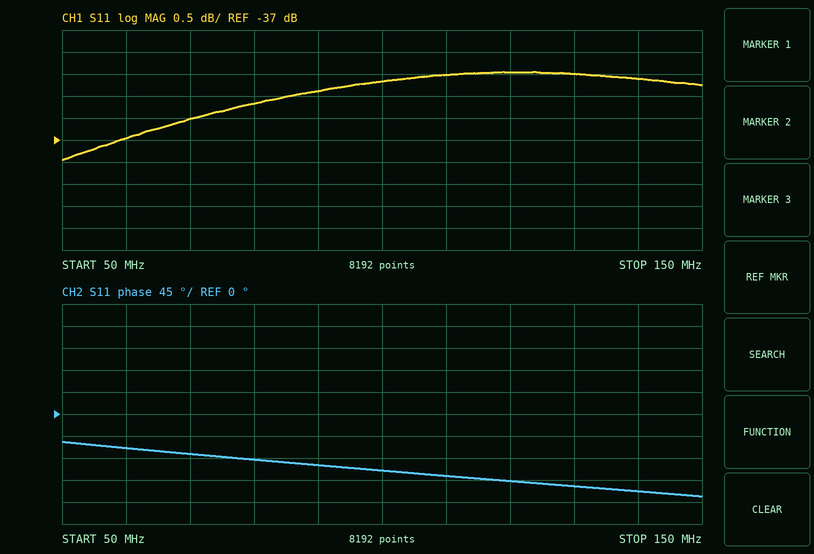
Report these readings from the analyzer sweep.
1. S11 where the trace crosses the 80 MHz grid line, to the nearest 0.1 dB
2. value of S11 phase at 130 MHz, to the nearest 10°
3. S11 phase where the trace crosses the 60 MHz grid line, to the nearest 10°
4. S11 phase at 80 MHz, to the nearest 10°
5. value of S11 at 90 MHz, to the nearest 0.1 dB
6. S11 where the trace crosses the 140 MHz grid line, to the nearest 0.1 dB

-36.2 dB
-150°
-70°
-90°
-35.9 dB
-35.6 dB
